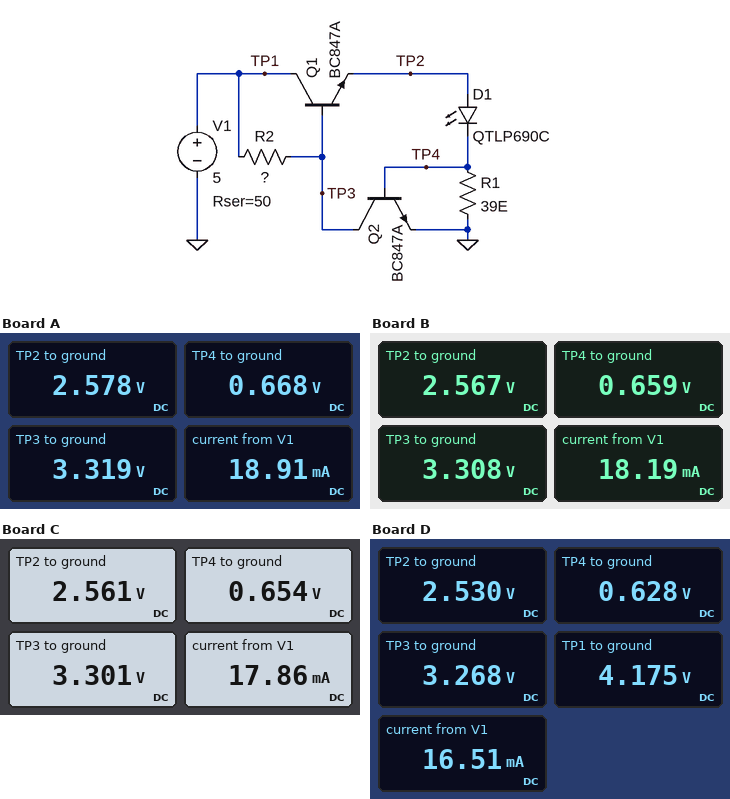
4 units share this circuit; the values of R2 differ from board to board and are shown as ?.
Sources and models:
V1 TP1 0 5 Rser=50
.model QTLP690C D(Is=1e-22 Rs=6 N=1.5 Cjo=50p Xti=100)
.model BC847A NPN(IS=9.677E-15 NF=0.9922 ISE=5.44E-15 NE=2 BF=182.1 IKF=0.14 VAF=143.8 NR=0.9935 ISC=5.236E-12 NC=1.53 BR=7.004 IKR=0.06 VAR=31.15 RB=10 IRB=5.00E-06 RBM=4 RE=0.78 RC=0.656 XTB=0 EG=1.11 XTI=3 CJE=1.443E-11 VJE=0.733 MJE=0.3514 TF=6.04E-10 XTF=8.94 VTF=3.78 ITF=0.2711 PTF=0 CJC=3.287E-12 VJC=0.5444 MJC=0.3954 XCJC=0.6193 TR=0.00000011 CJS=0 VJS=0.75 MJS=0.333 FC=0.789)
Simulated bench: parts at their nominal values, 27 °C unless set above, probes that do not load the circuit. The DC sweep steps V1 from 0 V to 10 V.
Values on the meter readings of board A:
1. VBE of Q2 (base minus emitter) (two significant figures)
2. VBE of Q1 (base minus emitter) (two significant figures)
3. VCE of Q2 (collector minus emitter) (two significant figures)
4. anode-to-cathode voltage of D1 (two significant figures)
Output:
670 mV
740 mV
3.3 V
1.9 V
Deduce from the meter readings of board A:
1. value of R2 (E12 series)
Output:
390 Ω
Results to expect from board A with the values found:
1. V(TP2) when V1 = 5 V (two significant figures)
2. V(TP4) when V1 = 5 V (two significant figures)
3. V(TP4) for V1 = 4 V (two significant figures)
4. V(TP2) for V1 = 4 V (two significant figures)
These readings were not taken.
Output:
2.6 V
670 mV
580 mV
2.5 V
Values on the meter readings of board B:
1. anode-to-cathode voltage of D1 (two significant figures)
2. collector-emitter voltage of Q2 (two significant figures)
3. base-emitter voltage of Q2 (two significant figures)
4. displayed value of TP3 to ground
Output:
1.9 V
3.3 V
660 mV
3.308 V
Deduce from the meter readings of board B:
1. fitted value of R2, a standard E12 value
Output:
560 Ω
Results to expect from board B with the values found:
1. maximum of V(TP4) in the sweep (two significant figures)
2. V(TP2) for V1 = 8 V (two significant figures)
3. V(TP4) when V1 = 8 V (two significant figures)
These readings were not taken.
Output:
720 mV
2.6 V
700 mV
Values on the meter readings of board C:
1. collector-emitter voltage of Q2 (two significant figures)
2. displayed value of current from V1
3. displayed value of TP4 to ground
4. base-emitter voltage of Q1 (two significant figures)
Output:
3.3 V
17.86 mA
0.654 V
740 mV
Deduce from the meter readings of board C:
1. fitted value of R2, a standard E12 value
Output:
680 Ω
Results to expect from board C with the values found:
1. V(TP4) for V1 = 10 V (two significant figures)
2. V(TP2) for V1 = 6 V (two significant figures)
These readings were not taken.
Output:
710 mV
2.6 V
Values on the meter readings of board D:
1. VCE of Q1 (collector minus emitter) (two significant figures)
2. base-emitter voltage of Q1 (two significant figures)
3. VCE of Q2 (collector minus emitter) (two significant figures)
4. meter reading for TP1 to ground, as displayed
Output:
1.6 V
740 mV
3.3 V
4.175 V
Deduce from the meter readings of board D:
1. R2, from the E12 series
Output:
1.8 kΩ
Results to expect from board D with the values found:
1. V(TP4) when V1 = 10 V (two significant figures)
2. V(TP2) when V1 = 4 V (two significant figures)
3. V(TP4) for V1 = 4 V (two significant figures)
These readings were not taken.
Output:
680 mV
2.4 V
530 mV
